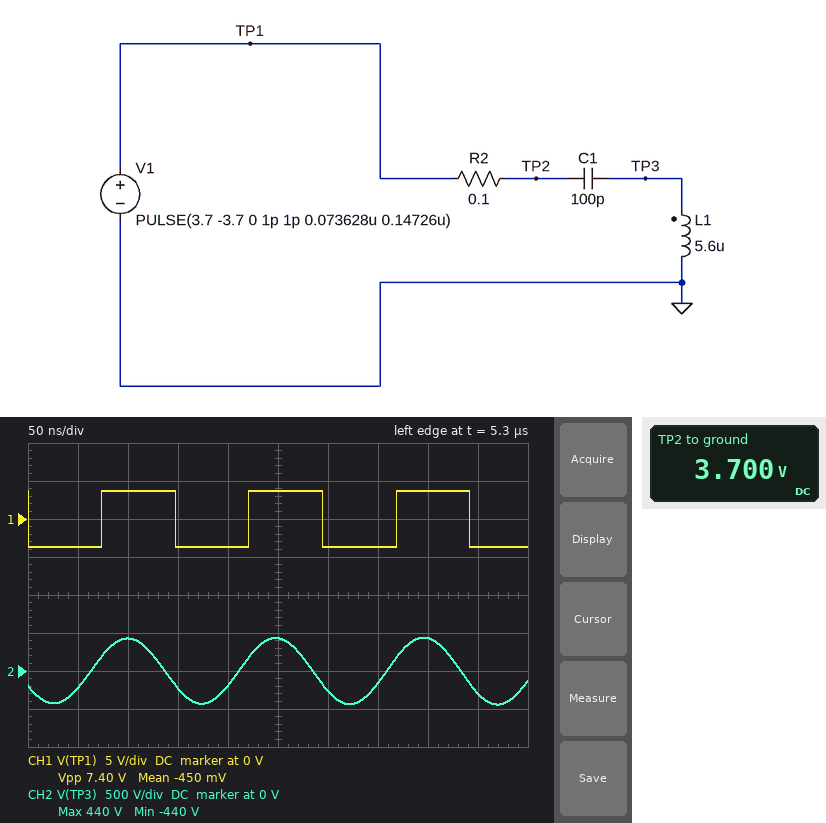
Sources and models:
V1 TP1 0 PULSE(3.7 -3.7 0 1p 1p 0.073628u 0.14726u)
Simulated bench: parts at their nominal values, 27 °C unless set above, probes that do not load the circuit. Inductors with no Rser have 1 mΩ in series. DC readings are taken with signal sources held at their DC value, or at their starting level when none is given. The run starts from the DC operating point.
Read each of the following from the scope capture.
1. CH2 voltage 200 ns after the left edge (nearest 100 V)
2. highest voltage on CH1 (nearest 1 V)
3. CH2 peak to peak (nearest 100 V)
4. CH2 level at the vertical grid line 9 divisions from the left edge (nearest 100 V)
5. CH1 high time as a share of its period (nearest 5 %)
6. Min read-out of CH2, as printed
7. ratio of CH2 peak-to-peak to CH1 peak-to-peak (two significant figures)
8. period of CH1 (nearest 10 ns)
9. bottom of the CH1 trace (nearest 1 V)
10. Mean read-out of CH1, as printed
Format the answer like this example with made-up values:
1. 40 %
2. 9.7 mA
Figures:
1. -200 V
2. 4 V
3. 900 V
4. -300 V
5. 50 %
6. -440 V
7. 120
8. 150 ns
9. -4 V
10. -450 mV
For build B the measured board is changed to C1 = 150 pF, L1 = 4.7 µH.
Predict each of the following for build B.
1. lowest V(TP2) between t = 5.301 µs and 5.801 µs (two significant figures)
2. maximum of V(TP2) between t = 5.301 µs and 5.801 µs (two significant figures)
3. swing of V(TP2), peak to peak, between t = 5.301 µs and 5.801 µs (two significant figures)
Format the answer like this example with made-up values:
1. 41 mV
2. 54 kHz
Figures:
1. -3.7 V
2. 3.7 V
3. 7.4 V
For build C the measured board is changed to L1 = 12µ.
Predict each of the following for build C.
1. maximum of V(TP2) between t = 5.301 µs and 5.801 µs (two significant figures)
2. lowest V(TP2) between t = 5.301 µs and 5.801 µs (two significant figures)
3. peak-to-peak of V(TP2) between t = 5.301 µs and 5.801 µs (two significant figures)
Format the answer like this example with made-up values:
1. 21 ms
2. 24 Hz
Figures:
1. 3.7 V
2. -3.7 V
3. 7.4 V
